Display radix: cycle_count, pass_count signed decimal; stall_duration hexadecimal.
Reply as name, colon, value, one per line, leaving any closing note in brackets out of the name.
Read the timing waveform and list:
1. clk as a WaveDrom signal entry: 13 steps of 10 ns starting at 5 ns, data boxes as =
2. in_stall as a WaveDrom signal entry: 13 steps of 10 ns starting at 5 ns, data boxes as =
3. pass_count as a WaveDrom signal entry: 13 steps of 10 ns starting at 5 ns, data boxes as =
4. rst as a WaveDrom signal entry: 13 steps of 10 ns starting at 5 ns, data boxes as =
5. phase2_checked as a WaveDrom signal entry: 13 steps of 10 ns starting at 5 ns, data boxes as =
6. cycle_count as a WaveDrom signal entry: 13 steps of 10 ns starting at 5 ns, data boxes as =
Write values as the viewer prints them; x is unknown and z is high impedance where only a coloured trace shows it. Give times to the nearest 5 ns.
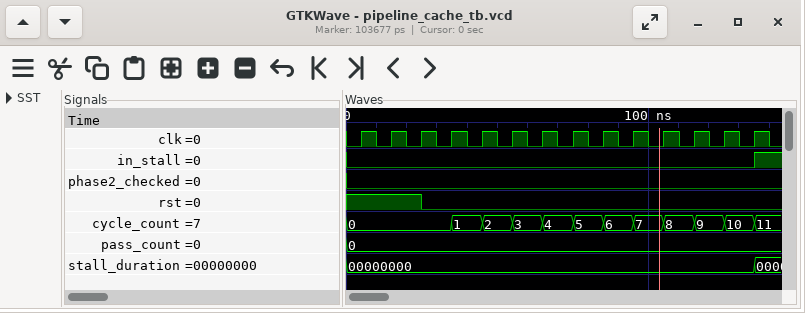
clk as a WaveDrom signal entry: 13 steps of 10 ns starting at 5 ns, data boxes as =: {name: 'clk', wave: 'p............'}
in_stall as a WaveDrom signal entry: 13 steps of 10 ns starting at 5 ns, data boxes as =: {name: 'in_stall', wave: '0............'}
pass_count as a WaveDrom signal entry: 13 steps of 10 ns starting at 5 ns, data boxes as =: {name: 'pass_count', wave: '=............', data: '0'}
rst as a WaveDrom signal entry: 13 steps of 10 ns starting at 5 ns, data boxes as =: {name: 'rst', wave: '1.0..........'}
phase2_checked as a WaveDrom signal entry: 13 steps of 10 ns starting at 5 ns, data boxes as =: {name: 'phase2_checked', wave: '0............'}
cycle_count as a WaveDrom signal entry: 13 steps of 10 ns starting at 5 ns, data boxes as =: {name: 'cycle_count', wave: '=..==========', data: '0 1 2 3 4 5 6 7 8 9 10'}
